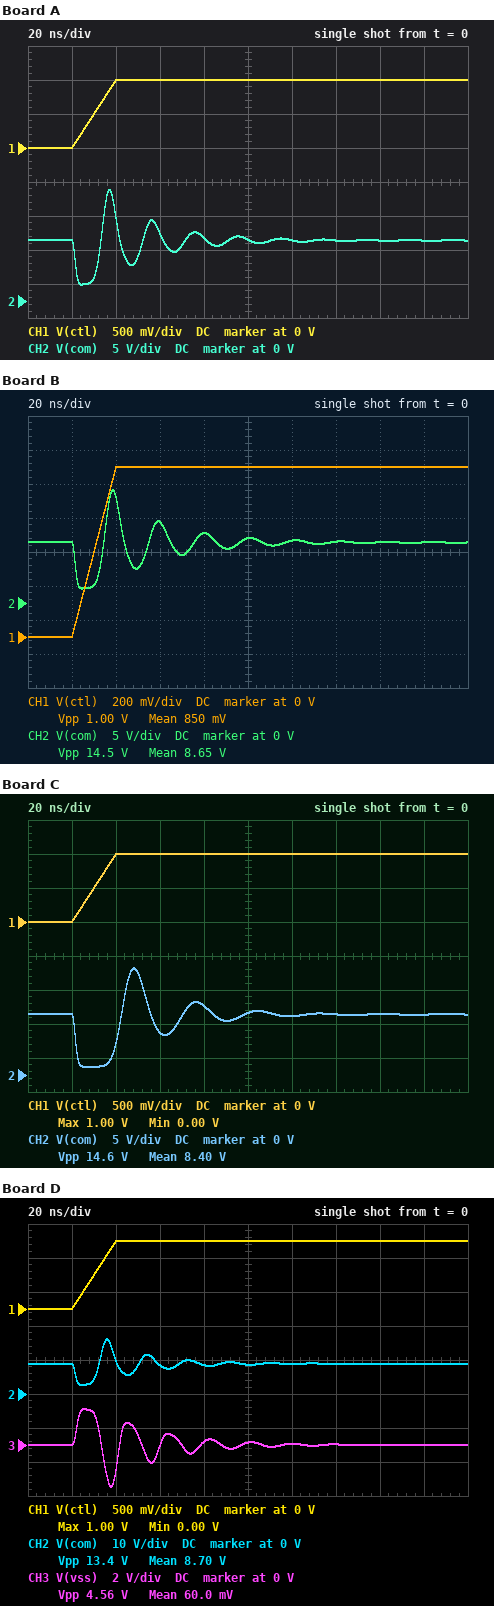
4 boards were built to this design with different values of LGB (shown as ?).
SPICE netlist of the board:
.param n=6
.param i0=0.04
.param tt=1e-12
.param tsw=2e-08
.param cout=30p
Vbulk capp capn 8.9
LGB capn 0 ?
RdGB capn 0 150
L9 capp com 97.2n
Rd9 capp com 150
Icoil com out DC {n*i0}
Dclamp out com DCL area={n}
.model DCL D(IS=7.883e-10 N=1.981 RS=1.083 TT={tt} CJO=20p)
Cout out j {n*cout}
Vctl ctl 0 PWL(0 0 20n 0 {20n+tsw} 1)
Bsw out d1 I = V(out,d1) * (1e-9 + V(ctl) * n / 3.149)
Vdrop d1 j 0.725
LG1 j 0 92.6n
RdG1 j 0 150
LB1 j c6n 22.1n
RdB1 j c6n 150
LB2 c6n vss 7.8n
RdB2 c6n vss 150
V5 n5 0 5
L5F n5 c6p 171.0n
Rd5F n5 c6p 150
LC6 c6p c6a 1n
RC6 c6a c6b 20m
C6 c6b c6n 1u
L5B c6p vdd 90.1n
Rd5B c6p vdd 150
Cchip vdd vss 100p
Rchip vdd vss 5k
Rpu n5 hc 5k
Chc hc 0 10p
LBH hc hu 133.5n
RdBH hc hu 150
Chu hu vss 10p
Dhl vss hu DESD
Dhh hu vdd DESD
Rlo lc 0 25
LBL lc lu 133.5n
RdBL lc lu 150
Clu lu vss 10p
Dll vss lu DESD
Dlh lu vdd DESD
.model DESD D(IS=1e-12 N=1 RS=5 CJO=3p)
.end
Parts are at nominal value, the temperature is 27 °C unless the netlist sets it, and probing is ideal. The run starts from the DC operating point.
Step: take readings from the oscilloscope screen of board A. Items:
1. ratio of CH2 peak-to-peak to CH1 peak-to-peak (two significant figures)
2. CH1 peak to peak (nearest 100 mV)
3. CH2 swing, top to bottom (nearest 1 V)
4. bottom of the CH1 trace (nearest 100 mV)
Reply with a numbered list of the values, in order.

1. 14
2. 1.0 V
3. 14 V
4. 0 V
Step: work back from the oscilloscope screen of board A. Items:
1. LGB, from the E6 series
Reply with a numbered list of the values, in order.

1. 68 nH
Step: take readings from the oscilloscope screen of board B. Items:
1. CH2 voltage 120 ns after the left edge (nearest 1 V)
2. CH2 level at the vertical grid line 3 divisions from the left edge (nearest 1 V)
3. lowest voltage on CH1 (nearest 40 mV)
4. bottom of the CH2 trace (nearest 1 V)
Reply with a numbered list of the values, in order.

1. 9 V
2. 12 V
3. 0 V
4. 2 V
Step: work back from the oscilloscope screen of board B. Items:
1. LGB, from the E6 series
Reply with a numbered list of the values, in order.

1. 100 nH
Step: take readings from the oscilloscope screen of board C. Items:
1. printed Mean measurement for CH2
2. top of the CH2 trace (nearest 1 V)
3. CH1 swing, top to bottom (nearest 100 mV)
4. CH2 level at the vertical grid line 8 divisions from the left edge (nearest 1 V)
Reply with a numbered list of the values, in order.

1. 8.40 V
2. 16 V
3. 1.0 V
4. 9 V
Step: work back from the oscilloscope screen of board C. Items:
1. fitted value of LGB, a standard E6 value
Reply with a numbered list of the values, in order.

1. 330 nH
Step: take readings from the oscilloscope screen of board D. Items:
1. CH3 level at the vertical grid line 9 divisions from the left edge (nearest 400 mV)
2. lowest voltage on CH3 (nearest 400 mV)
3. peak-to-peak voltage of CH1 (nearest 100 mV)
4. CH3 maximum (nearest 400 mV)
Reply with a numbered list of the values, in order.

1. 0 V
2. -2.4 V
3. 1.0 V
4. 2.0 V
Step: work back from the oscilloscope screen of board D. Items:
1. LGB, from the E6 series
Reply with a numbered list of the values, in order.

1. 47 nH
